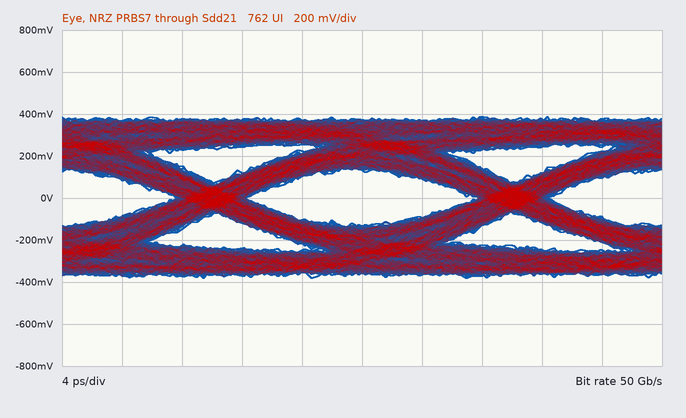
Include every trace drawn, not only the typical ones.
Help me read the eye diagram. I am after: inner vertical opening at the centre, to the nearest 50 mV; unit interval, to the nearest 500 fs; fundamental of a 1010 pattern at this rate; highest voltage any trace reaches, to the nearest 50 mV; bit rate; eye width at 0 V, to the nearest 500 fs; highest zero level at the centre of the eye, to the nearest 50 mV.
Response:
250 mV
20.0 ps
25 GHz
400 mV
50 Gb/s
15.5 ps
-150 mV
